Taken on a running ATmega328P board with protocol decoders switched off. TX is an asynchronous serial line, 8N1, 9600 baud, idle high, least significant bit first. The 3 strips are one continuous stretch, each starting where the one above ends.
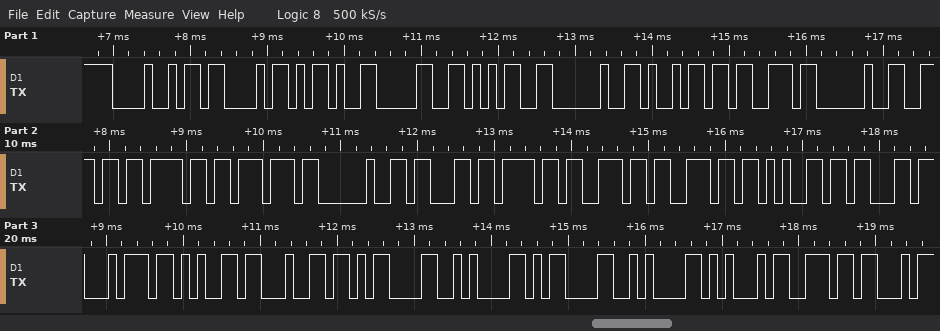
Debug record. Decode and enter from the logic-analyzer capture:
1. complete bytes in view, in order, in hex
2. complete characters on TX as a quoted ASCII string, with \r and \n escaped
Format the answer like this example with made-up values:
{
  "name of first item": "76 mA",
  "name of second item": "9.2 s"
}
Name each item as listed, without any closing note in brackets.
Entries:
{
  "complete bytes in view, in order, in hex": "0x48 0x43 0x2D 0x30 0x35 0x20 0x69 0x73 0x20 0x6E 0x6F 0x77 0x20 0x63 0x6F 0x6E 0x6E 0x65 0x63 0x74 0x65 0x64 0x0D 0x0A 0x0D 0x0A 0x45 0x6E",
  "complete characters on TX as a quoted ASCII string, with \\r and \\n escaped": "\"HC-05 is now connected\\r\\n\\r\\nEn\""
}
